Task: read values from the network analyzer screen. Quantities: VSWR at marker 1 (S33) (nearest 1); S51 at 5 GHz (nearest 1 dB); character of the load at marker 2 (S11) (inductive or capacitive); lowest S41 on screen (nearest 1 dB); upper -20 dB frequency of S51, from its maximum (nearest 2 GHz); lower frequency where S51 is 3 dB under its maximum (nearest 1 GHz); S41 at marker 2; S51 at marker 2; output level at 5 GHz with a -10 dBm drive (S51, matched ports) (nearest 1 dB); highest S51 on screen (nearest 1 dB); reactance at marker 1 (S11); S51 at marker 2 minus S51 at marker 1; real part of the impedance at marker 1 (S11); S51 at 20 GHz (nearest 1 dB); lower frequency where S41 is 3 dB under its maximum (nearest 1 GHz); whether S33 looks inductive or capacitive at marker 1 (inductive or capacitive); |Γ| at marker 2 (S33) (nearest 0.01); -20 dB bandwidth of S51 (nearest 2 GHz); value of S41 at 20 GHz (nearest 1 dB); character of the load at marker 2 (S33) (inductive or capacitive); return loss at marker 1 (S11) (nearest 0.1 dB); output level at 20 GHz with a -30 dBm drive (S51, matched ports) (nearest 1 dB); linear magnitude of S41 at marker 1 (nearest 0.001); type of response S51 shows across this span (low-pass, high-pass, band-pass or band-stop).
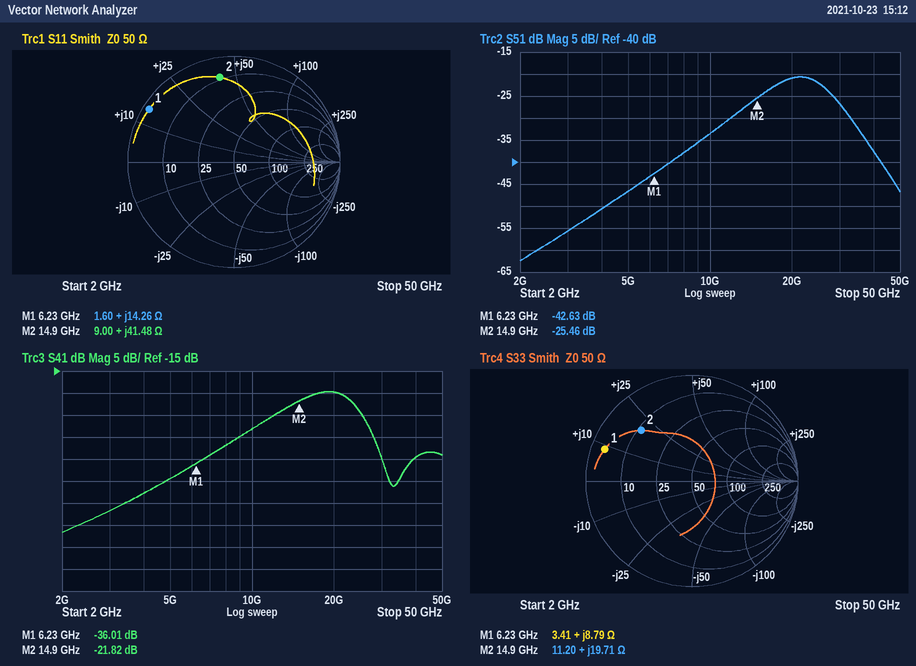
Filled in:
15
-47 dB
inductive
-52 dB
44 GHz
16 GHz
-21.82 dB
-25.46 dB
-57 dBm
-21 dB
+14.26 Ω
17.17 dB
1.60 Ω
-21 dB
14 GHz
inductive
0.68
36 GHz
-20 dB
inductive
0.5 dB
-51 dBm
0.016
band-pass
